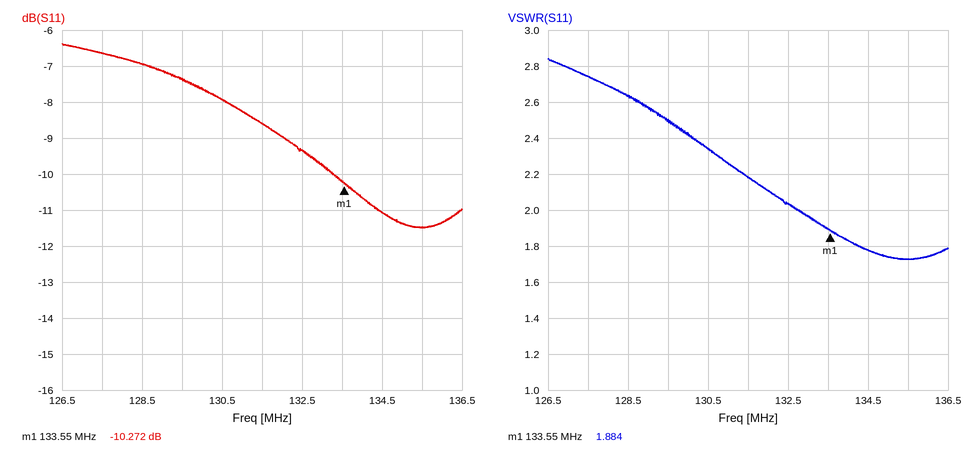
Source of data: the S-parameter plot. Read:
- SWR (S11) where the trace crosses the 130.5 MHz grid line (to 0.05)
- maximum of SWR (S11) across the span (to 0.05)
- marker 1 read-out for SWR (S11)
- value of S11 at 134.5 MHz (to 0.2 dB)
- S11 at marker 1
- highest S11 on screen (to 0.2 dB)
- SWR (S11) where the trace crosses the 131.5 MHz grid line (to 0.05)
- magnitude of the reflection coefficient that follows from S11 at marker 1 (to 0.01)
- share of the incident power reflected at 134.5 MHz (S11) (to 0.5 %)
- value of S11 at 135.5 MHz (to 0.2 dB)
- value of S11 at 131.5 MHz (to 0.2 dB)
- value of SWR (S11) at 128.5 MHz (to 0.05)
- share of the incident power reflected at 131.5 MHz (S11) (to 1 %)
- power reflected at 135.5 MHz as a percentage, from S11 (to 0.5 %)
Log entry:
2.35
2.85
1.884
-11.0 dB
-10.272 dB
-6.4 dB
2.20
0.31
8.0 %
-11.4 dB
-8.6 dB
2.65
14 %
7.0 %
